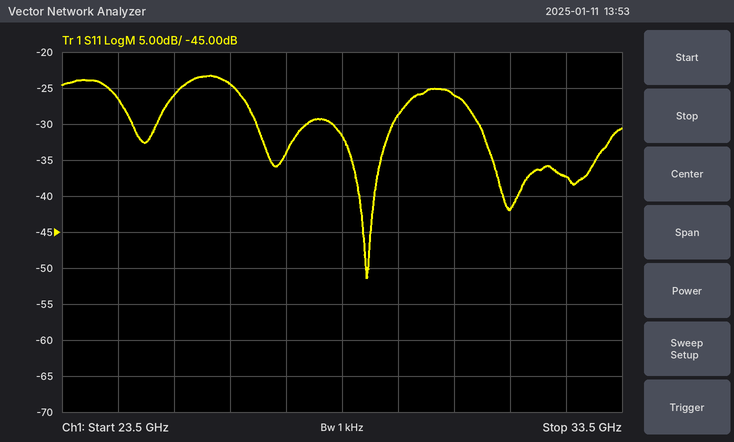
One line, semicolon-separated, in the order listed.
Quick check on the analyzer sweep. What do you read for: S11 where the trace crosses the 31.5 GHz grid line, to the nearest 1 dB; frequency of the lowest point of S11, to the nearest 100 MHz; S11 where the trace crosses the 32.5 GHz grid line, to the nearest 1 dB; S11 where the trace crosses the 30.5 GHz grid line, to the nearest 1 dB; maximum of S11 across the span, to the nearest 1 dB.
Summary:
-42 dB; 28.9 GHz; -37 dB; -26 dB; -23 dB
